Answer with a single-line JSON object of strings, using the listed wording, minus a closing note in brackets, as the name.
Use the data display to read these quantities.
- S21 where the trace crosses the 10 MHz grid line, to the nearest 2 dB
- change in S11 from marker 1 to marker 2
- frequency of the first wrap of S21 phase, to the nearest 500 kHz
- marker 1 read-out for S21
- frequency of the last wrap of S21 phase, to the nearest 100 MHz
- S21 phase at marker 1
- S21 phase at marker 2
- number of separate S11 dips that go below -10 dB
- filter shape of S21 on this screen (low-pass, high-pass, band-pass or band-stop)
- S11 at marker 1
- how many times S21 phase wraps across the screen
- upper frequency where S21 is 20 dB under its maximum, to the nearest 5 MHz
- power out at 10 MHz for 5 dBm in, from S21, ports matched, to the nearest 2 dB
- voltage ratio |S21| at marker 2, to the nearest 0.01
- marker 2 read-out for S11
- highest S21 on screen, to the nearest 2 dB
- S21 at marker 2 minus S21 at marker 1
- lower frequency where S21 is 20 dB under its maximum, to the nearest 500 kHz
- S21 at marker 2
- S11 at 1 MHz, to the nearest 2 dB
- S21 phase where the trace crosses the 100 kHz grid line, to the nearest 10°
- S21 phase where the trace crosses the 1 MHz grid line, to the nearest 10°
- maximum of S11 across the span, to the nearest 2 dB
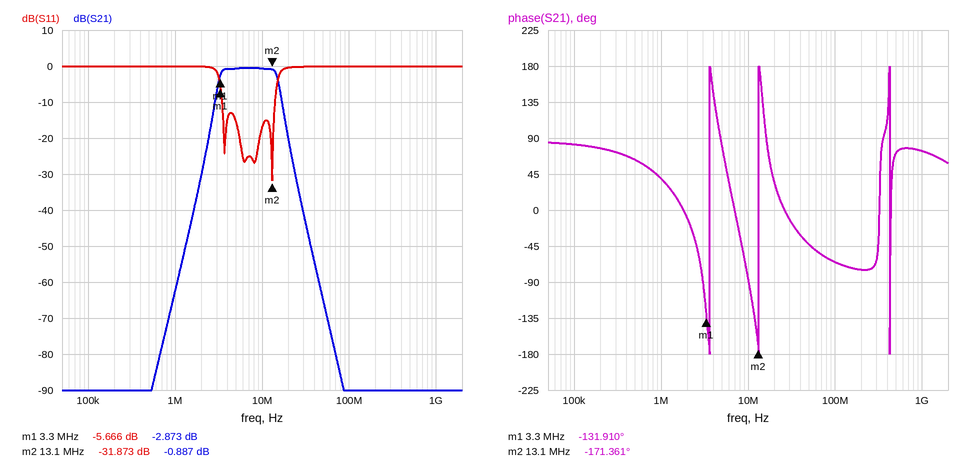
{"S21 where the trace crosses the 10 MHz grid line, to the nearest 2 dB": "0 dB", "change in S11 from marker 1 to marker 2": "-26.207 dB", "frequency of the first wrap of S21 phase, to the nearest 500 kHz": "3.5 MHz", "marker 1 read-out for S21": "-2.873 dB", "frequency of the last wrap of S21 phase, to the nearest 100 MHz": "400 MHz", "S21 phase at marker 1": "-131.910°", "S21 phase at marker 2": "-171.361°", "number of separate S11 dips that go below -10 dB": "3", "filter shape of S21 on this screen": "band-pass", "S11 at marker 1": "-5.666 dB", "how many times S21 phase wraps across the screen": "3", "upper frequency where S21 is 20 dB under its maximum, to the nearest 5 MHz": "20 MHz", "power out at 10 MHz for 5 dBm in, from S21, ports matched, to the nearest 2 dB": "4 dBm", "voltage ratio |S21| at marker 2, to the nearest 0.01": "0.90", "marker 2 read-out for S11": "-31.873 dB", "highest S21 on screen, to the nearest 2 dB": "0 dB", "S21 at marker 2 minus S21 at marker 1": "1.986 dB", "lower frequency where S21 is 20 dB under its maximum, to the nearest 500 kHz": "2.5 MHz", "S21 at marker 2": "-0.887 dB", "S11 at 1 MHz, to the nearest 2 dB": "0 dB", "S21 phase where the trace crosses the 100 kHz grid line, to the nearest 10°": "80°", "S21 phase where the trace crosses the 1 MHz grid line, to the nearest 10°": "40°", "maximum of S11 across the span, to the nearest 2 dB": "0 dB"}
